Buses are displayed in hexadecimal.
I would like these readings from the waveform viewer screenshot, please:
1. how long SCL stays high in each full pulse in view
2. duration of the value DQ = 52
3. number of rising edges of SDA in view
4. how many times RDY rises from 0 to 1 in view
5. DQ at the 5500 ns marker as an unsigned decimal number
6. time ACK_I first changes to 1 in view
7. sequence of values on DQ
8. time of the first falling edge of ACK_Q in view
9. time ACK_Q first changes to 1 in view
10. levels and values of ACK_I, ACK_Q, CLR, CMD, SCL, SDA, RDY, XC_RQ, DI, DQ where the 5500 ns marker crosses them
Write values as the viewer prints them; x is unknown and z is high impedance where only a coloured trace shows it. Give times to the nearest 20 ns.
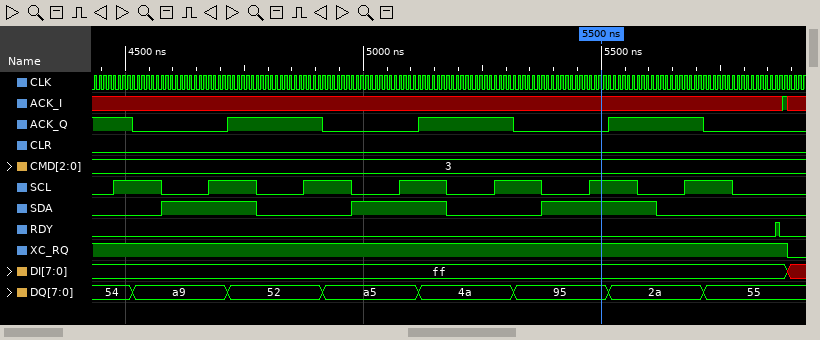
100 ns, 100 ns, 100 ns, 100 ns, 100 ns, 100 ns, 100 ns
200 ns
3
1
149
5880 ns
54, a9, 52, a5, 4a, 95, 2a, 55
4520 ns
4720 ns
ACK_I=x, ACK_Q=0, CLR=0, CMD=3, SCL=1, SDA=1, RDY=0, XC_RQ=1, DI=ff, DQ=95
